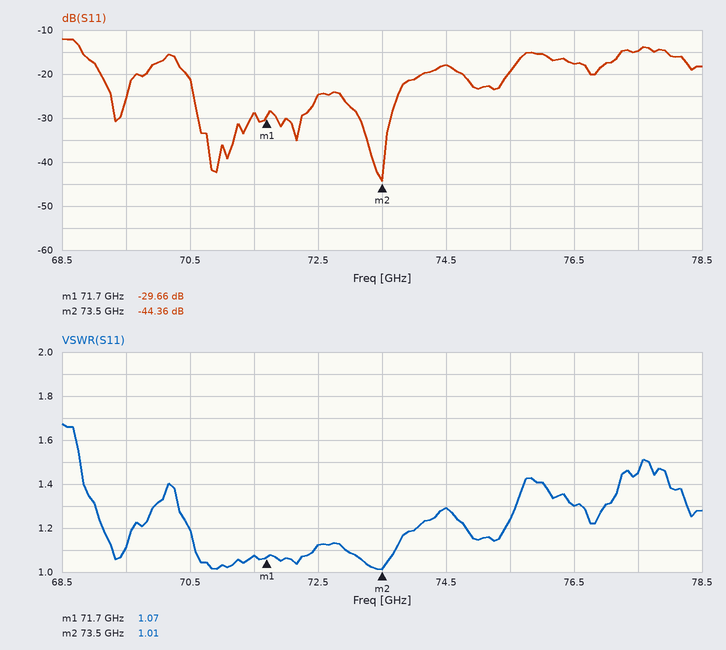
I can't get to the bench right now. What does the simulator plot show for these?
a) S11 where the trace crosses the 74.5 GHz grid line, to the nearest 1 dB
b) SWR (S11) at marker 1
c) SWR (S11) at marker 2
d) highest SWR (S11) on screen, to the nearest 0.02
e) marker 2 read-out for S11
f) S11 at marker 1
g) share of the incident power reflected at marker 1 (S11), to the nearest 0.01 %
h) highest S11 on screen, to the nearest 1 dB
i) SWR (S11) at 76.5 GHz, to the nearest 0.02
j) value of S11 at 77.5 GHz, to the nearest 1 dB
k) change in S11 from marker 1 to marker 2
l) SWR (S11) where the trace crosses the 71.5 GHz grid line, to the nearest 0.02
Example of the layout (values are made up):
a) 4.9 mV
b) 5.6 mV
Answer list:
a) -18 dB
b) 1.07
c) 1.01
d) 1.68
e) -44.36 dB
f) -29.66 dB
g) 0.11 %
h) -12 dB
i) 1.30
j) -15 dB
k) -14.70 dB
l) 1.08
